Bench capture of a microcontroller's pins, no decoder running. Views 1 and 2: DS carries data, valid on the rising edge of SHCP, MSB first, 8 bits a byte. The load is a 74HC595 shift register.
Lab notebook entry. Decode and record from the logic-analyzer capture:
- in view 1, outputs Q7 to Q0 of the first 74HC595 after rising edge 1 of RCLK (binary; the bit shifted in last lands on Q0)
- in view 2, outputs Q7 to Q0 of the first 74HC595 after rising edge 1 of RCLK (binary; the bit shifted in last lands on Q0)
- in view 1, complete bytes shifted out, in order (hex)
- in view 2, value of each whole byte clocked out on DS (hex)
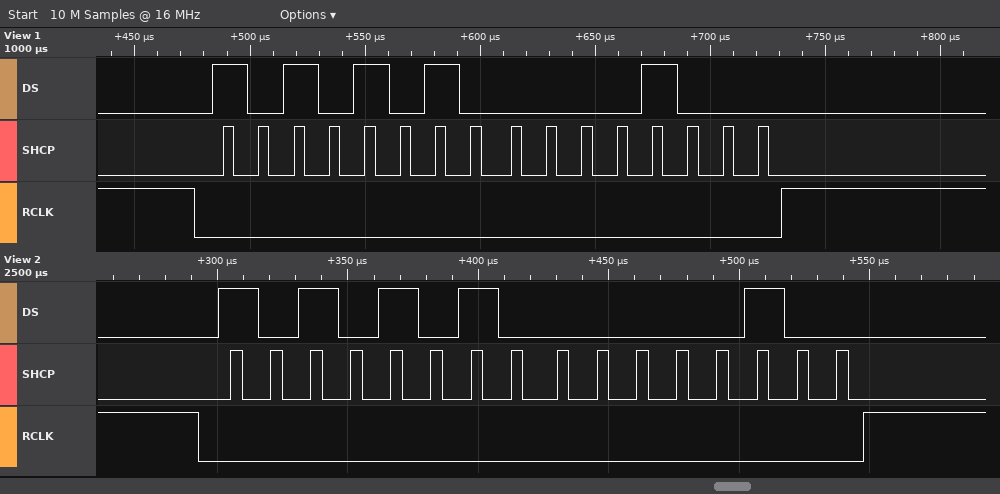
00001000
00000100
AA 08
AA 04
